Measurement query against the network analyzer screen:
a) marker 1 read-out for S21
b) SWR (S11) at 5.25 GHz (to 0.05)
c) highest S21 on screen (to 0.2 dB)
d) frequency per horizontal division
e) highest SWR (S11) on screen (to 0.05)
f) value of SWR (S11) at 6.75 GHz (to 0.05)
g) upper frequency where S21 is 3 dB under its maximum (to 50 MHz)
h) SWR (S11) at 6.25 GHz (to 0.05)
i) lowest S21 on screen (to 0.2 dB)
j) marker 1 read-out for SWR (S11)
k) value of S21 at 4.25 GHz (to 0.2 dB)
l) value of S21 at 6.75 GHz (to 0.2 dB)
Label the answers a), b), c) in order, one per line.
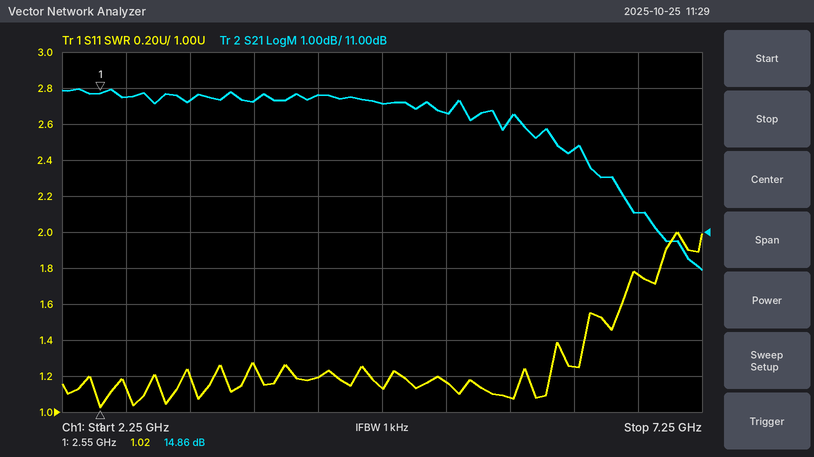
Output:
a) 14.86 dB
b) 1.15
c) 15.0 dB
d) 500 MHz
e) 2.00
f) 1.75
g) 6.65 GHz
h) 1.25
i) 10.0 dB
j) 1.02
k) 14.8 dB
l) 11.6 dB
